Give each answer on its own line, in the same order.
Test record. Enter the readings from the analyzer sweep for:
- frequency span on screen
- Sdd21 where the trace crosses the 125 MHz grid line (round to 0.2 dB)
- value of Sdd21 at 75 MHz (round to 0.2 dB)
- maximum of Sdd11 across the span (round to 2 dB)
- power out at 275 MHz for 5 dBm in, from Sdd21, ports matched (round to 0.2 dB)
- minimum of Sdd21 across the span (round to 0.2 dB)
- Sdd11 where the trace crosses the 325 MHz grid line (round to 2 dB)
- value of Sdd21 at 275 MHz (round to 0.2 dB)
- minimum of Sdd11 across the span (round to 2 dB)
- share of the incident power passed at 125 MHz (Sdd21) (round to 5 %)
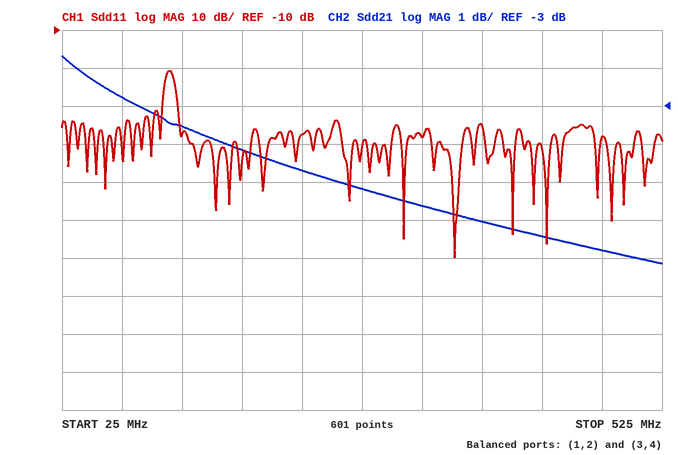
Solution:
500 MHz
-3.6 dB
-2.8 dB
-20 dB
-0.2 dBm
-7.2 dB
-38 dB
-5.2 dB
-70 dB
45 %
